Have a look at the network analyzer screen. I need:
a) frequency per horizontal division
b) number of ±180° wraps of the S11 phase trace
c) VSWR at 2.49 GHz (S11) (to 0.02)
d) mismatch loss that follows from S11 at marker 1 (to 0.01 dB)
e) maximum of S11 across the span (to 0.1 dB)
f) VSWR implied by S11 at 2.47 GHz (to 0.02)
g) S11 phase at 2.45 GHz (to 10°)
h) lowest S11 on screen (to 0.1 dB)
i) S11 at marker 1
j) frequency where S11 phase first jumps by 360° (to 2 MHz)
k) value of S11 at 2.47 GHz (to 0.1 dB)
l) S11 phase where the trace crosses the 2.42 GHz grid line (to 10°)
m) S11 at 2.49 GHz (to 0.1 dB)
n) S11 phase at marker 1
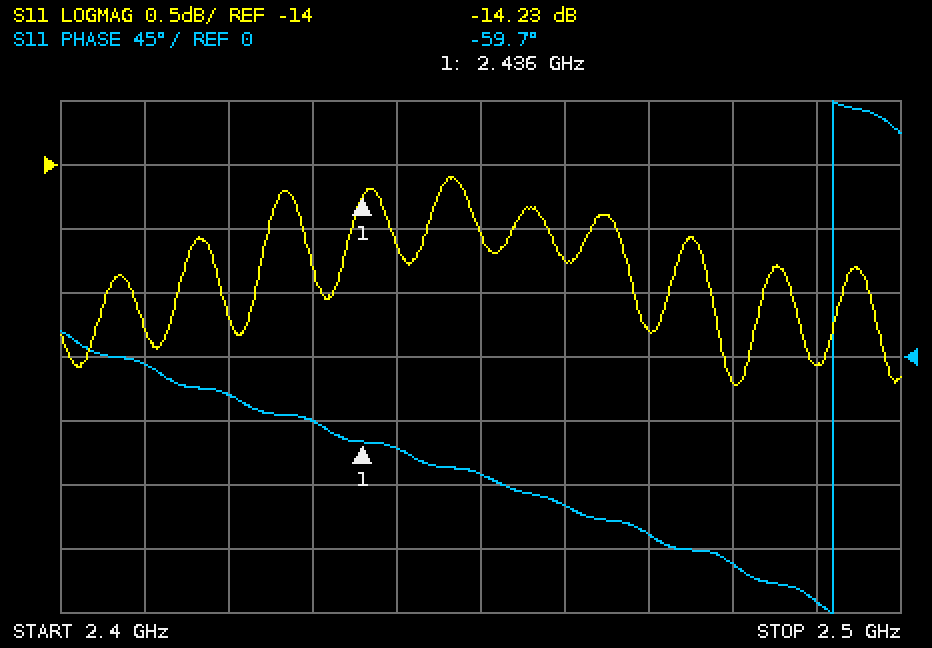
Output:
10 MHz
1
1.40
0.17 dB
-14.1 dB
1.42
-80°
-15.7 dB
-14.23 dB
2.492 GHz
-15.3 dB
-30°
-15.6 dB
-59.7°
